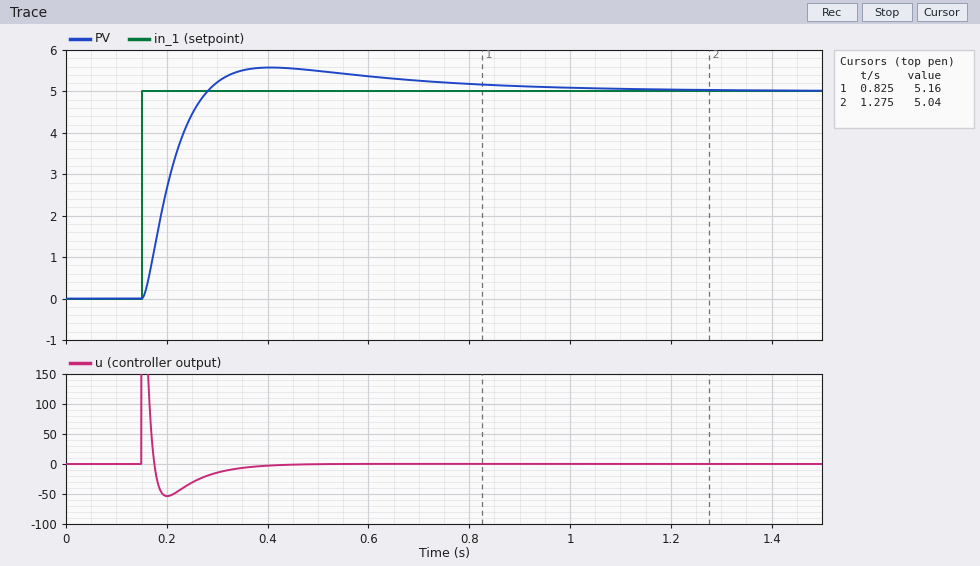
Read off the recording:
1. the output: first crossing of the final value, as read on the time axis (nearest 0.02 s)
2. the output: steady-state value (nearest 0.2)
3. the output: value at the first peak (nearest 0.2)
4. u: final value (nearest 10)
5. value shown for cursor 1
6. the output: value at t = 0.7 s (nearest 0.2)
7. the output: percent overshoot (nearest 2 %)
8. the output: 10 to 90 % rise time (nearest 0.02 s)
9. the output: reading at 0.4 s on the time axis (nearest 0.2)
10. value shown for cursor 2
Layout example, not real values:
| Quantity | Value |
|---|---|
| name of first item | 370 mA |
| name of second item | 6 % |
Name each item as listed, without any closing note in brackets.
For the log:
| Quantity | Value |
|---|---|
| the output: first crossing of the final value, as read on the time axis | 0.28 s |
| the output: steady-state value | 5.0 |
| the output: value at the first peak | 5.6 |
| u: final value | 0 |
| value shown for cursor 1 | 5.16 |
| the output: value at t = 0.7 s | 5.2 |
| the output: percent overshoot | 12 % |
| the output: 10 to 90 % rise time | 0.08 s |
| the output: reading at 0.4 s on the time axis | 5.6 |
| value shown for cursor 2 | 5.04 |
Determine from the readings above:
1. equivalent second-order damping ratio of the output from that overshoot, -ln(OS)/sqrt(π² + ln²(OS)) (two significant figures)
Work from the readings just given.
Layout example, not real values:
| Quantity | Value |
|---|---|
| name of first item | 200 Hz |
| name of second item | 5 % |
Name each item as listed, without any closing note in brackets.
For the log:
| Quantity | Value |
|---|---|
| equivalent second-order damping ratio of the output from that overshoot, -ln(OS)/sqrt(π² + ln²(OS)) | 0.56 |
